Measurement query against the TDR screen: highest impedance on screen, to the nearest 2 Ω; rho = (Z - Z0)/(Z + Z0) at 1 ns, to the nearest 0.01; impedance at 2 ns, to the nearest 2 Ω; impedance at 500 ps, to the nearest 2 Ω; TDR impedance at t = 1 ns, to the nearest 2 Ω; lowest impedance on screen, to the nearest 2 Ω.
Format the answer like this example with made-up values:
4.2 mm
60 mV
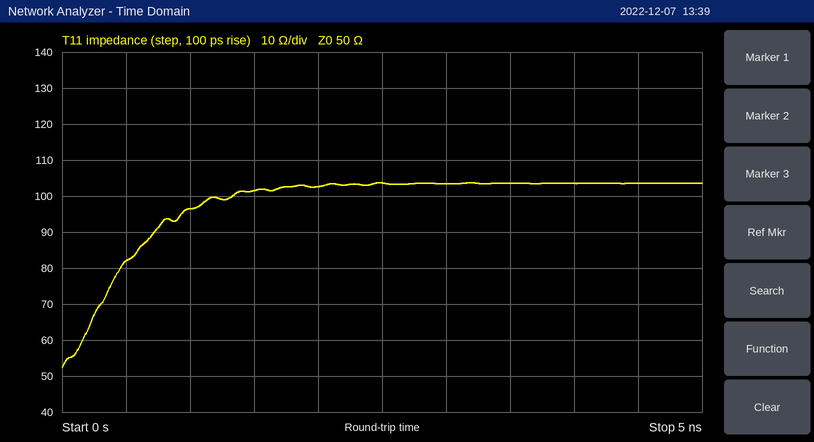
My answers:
104 Ω
+0.32
102 Ω
82 Ω
96 Ω
52 Ω
